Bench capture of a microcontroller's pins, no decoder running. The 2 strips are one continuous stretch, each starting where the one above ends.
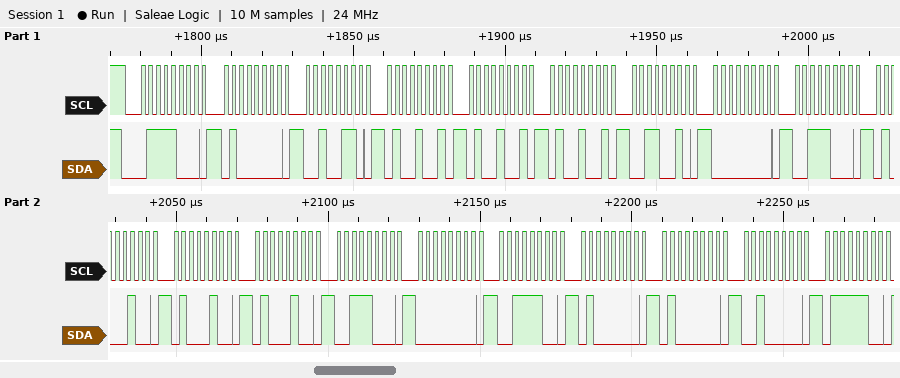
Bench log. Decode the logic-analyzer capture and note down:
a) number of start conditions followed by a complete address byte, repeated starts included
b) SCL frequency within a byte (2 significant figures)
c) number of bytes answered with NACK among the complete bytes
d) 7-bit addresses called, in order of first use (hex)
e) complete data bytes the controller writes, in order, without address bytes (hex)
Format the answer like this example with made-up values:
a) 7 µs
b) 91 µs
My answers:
a) 1
b) 400 kHz
c) 0
d) 0x3C
e) 40 26 49 49 49 32 00 38 44 44 44 38 00 3C 40 40 20 7C
